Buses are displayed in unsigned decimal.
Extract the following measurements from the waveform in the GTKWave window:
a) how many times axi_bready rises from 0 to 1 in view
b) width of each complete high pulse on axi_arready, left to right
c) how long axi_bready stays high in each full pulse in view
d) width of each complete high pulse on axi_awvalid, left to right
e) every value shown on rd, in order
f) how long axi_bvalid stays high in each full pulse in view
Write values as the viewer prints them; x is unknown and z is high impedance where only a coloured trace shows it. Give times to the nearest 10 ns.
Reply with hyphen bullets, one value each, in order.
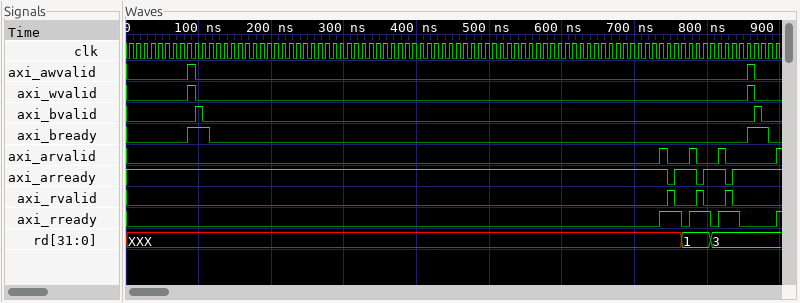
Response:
- 2
- 30 ns, 30 ns
- 30 ns, 30 ns
- 10 ns, 10 ns
- XXX, 1, 3
- 10 ns, 10 ns
